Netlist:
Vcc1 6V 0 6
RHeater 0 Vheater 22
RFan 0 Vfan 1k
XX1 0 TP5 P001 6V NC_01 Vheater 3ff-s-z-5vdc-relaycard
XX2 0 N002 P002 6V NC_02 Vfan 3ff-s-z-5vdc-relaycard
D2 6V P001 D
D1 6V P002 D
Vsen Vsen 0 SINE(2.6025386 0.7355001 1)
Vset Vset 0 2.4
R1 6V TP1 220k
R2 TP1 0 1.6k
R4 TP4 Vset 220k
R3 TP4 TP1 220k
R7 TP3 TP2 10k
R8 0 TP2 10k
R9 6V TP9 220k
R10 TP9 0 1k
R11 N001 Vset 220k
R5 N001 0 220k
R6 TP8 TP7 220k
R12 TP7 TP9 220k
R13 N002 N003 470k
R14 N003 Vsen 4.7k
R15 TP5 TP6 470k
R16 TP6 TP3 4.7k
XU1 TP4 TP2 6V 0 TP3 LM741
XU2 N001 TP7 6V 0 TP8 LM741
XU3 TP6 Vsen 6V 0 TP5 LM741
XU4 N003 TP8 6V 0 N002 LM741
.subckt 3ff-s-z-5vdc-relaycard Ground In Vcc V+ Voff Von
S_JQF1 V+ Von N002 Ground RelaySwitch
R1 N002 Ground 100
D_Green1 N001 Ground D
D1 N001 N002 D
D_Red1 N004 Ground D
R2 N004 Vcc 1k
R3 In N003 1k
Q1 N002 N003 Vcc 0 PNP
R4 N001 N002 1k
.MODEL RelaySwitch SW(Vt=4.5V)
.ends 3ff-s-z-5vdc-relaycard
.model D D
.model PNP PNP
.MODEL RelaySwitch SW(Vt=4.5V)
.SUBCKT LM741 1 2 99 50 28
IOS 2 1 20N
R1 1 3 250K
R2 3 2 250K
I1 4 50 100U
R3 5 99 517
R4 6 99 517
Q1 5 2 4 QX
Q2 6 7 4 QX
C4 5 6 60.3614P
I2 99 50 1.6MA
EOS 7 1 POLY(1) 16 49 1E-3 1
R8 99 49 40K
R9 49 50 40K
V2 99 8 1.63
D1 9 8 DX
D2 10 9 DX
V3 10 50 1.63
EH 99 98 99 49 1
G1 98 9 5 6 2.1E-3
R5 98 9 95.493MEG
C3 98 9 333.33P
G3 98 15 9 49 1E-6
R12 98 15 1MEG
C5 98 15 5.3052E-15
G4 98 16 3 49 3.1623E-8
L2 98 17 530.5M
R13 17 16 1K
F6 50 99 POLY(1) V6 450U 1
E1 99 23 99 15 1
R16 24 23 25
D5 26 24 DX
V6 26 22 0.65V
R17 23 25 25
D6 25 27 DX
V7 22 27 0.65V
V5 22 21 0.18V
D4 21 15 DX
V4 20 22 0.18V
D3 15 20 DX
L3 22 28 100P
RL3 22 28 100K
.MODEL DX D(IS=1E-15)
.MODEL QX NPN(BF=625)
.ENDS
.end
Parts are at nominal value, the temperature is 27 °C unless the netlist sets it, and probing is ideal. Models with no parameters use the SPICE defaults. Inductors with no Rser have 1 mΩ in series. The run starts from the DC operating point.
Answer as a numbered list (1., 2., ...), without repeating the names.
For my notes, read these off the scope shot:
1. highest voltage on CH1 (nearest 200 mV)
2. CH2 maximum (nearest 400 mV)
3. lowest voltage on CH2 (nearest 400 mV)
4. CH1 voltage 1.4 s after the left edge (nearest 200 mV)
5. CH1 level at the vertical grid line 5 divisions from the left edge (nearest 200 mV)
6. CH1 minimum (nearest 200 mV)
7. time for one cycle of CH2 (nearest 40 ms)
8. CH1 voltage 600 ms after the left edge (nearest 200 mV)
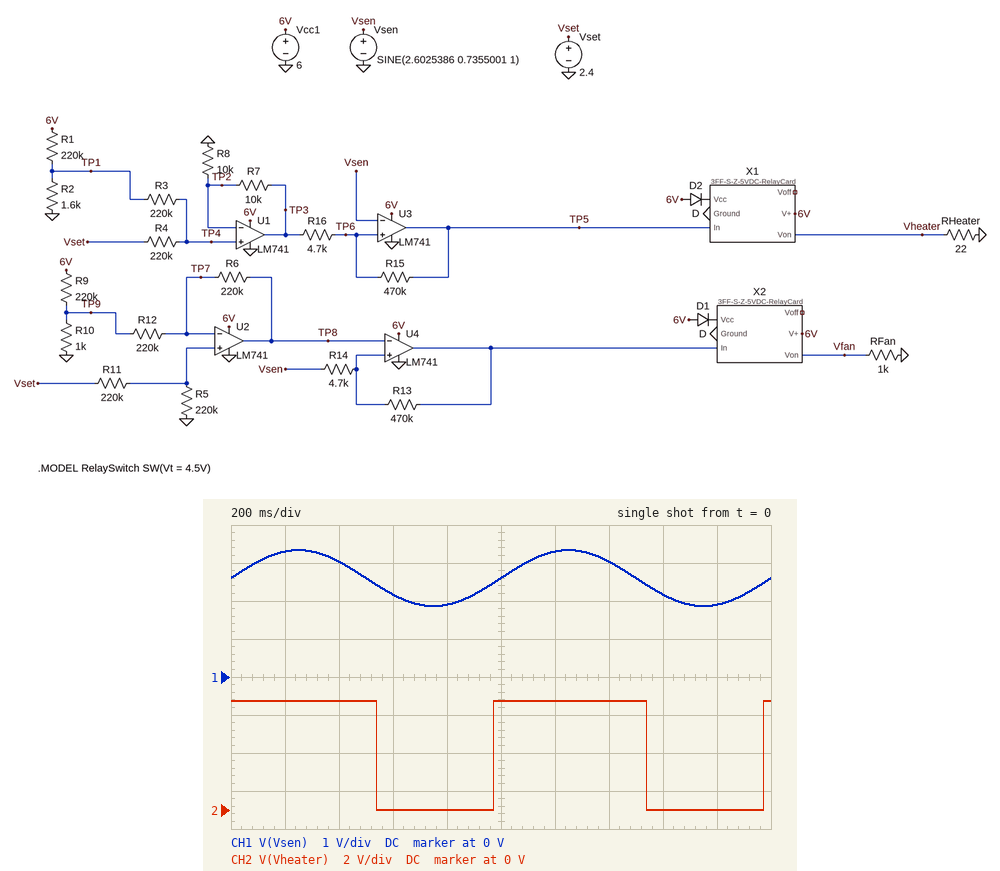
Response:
1. 3.4 V
2. 5.6 V
3. 0 V
4. 3.0 V
5. 2.6 V
6. 1.8 V
7. 1.00 s
8. 2.2 V
